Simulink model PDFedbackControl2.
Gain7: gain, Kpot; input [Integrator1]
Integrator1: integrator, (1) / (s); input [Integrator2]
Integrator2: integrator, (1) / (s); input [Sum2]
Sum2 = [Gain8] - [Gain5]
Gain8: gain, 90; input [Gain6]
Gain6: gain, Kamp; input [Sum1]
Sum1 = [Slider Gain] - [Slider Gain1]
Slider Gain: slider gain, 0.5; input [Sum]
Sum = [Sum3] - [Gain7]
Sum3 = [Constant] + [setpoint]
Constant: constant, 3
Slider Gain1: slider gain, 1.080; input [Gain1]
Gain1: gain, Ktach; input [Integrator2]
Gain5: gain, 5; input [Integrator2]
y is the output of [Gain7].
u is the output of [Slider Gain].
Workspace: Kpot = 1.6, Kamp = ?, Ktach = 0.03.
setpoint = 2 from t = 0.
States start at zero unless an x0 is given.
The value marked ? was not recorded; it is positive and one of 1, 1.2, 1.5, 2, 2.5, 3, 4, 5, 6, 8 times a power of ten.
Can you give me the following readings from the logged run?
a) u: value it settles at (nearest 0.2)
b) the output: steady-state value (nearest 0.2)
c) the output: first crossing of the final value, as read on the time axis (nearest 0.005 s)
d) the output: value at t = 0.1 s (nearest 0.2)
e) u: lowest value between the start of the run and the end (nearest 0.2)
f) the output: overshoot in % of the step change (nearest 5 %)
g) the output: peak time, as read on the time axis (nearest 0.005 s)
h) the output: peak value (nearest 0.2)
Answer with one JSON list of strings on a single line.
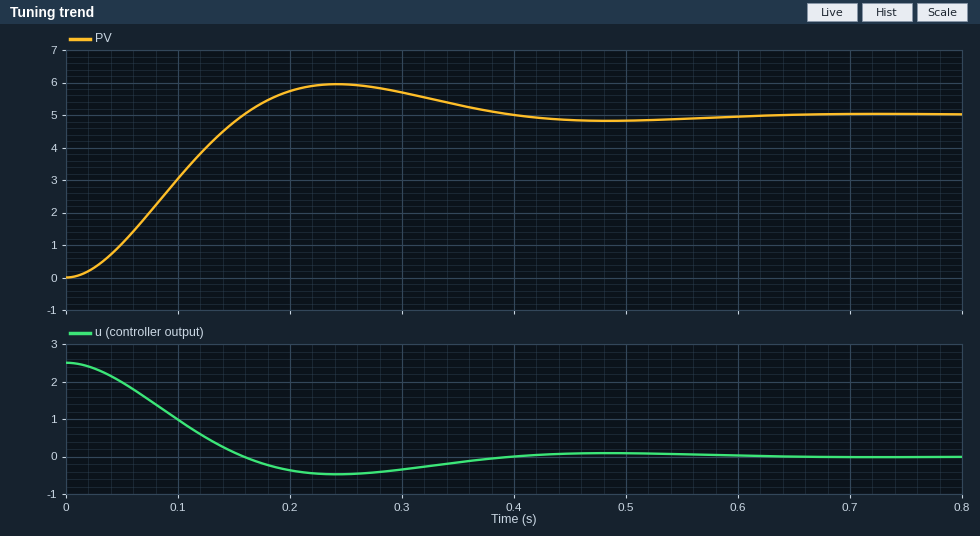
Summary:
["0.0", "5.0", "0.160 s", "3.0", "-0.4", "20 %", "0.240 s", "6.0"]
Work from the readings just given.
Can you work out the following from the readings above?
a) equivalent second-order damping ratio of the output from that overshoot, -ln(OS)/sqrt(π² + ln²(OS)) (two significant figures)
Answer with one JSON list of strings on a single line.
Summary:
["0.46"]
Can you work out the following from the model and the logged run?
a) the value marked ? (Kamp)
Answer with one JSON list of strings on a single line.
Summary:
["3"]
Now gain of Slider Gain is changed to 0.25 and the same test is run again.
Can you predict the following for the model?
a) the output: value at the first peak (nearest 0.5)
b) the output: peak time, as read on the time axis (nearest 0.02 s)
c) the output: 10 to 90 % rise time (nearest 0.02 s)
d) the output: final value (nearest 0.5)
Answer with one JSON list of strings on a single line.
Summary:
["5.5", "0.40 s", "0.20 s", "5.0"]
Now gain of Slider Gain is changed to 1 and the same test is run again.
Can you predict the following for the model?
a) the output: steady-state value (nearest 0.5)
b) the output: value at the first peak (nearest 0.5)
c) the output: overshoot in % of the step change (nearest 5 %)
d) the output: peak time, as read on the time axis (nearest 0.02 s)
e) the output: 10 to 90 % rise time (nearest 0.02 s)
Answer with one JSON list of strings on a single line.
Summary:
["5.0", "6.5", "35 %", "0.16 s", "0.06 s"]
